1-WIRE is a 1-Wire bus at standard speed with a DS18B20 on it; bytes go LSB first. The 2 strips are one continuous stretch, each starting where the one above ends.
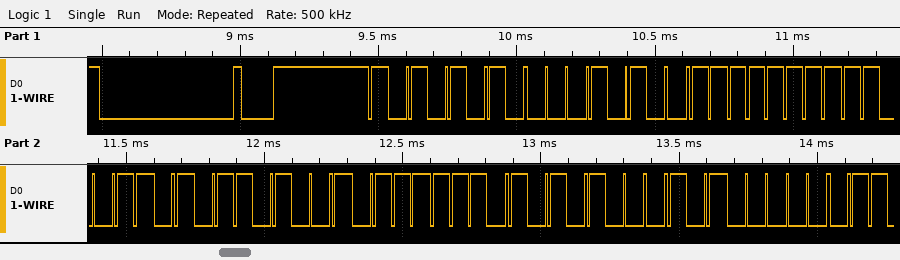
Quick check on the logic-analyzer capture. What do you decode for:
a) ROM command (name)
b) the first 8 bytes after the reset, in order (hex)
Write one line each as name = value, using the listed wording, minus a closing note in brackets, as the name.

ROM command = Match ROM
the first 8 bytes after the reset, in order = 55 28 FF B3 96 7E 15 05
